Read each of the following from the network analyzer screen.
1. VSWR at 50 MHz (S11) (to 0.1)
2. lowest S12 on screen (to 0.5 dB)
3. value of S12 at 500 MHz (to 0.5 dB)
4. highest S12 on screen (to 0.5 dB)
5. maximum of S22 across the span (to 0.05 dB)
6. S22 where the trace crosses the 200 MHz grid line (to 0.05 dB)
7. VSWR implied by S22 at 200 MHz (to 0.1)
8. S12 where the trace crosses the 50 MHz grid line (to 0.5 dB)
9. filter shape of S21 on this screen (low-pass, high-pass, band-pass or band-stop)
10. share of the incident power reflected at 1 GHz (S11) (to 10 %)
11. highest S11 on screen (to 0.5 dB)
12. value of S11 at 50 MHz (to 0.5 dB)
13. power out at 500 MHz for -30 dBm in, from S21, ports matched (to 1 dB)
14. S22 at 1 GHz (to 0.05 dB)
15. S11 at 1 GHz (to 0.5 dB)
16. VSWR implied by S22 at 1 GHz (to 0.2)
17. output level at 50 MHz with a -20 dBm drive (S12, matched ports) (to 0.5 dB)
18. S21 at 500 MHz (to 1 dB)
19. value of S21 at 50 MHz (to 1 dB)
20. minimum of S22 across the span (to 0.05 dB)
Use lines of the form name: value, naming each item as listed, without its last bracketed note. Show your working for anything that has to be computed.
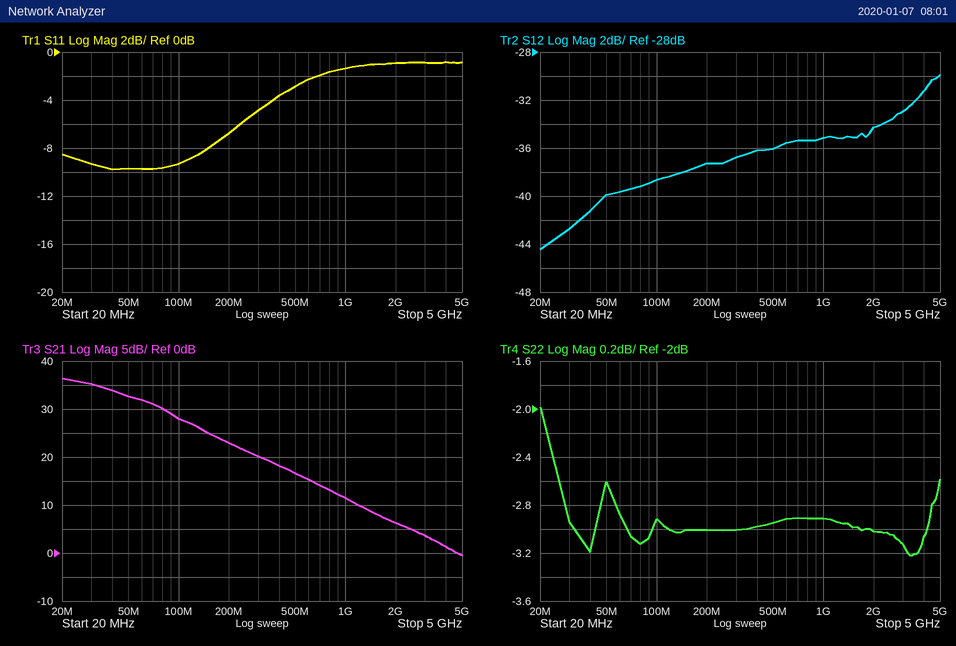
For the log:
VSWR at 50 MHz (S11): |Γ| = 10^(-9.5/20) = 0.3350; VSWR = (1 + 0.3350)/(1 − 0.3350) ≈ 2.0
lowest S12 on screen: -44.5 dB
value of S12 at 500 MHz: -36.0 dB
highest S12 on screen: -30.0 dB
maximum of S22 across the span: -2.00 dB
S22 where the trace crosses the 200 MHz grid line: -3.00 dB
VSWR implied by S22 at 200 MHz: |Γ| = 10^(-3/20) = 0.7079; VSWR = (1 + 0.7079)/(1 − 0.7079) ≈ 5.8
S12 where the trace crosses the 50 MHz grid line: -40.0 dB
filter shape of S21 on this screen: low-pass
share of the incident power reflected at 1 GHz (S11): 10^(-1.5/10) ≈ 70.8 %, so 70 % to the nearest 10 %
highest S11 on screen: -1.0 dB
value of S11 at 50 MHz: -9.5 dB
power out at 500 MHz for -30 dBm in, from S21, ports matched: -30 dBm + (17 dB) = -13 dBm
S22 at 1 GHz: -2.90 dB
S11 at 1 GHz: -1.5 dB
VSWR implied by S22 at 1 GHz: |Γ| = 10^(-2.9/20) = 0.7161; VSWR = (1 + 0.7161)/(1 − 0.7161) ≈ 6.0
output level at 50 MHz with a -20 dBm drive (S12, matched ports): -20 dBm + (-40.0 dB) = -60.0 dBm
S21 at 500 MHz: 17 dB
value of S21 at 50 MHz: 33 dB
minimum of S22 across the span: -3.20 dB
